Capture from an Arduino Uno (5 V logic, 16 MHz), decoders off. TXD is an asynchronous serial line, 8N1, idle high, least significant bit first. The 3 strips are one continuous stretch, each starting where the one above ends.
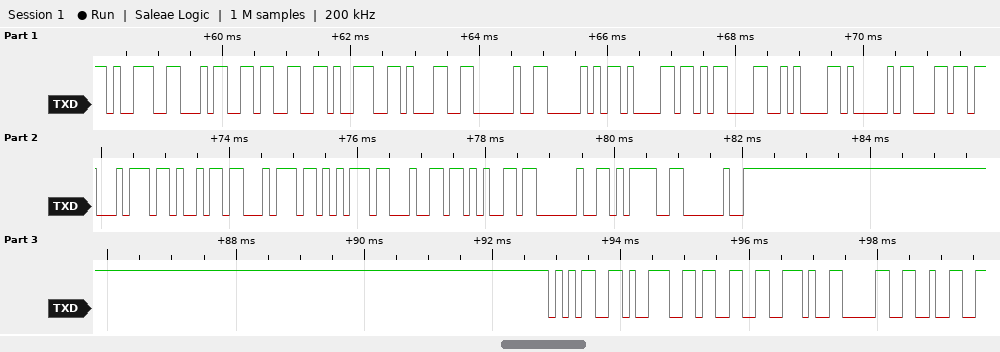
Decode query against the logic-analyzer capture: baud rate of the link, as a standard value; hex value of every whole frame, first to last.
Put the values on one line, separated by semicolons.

9600 baud; 39 34 33 39 31 20 50 61 0D 0A 41 6C 74 69 74 75 64 65 20 3D 20 35 39 33 2E 30 32
